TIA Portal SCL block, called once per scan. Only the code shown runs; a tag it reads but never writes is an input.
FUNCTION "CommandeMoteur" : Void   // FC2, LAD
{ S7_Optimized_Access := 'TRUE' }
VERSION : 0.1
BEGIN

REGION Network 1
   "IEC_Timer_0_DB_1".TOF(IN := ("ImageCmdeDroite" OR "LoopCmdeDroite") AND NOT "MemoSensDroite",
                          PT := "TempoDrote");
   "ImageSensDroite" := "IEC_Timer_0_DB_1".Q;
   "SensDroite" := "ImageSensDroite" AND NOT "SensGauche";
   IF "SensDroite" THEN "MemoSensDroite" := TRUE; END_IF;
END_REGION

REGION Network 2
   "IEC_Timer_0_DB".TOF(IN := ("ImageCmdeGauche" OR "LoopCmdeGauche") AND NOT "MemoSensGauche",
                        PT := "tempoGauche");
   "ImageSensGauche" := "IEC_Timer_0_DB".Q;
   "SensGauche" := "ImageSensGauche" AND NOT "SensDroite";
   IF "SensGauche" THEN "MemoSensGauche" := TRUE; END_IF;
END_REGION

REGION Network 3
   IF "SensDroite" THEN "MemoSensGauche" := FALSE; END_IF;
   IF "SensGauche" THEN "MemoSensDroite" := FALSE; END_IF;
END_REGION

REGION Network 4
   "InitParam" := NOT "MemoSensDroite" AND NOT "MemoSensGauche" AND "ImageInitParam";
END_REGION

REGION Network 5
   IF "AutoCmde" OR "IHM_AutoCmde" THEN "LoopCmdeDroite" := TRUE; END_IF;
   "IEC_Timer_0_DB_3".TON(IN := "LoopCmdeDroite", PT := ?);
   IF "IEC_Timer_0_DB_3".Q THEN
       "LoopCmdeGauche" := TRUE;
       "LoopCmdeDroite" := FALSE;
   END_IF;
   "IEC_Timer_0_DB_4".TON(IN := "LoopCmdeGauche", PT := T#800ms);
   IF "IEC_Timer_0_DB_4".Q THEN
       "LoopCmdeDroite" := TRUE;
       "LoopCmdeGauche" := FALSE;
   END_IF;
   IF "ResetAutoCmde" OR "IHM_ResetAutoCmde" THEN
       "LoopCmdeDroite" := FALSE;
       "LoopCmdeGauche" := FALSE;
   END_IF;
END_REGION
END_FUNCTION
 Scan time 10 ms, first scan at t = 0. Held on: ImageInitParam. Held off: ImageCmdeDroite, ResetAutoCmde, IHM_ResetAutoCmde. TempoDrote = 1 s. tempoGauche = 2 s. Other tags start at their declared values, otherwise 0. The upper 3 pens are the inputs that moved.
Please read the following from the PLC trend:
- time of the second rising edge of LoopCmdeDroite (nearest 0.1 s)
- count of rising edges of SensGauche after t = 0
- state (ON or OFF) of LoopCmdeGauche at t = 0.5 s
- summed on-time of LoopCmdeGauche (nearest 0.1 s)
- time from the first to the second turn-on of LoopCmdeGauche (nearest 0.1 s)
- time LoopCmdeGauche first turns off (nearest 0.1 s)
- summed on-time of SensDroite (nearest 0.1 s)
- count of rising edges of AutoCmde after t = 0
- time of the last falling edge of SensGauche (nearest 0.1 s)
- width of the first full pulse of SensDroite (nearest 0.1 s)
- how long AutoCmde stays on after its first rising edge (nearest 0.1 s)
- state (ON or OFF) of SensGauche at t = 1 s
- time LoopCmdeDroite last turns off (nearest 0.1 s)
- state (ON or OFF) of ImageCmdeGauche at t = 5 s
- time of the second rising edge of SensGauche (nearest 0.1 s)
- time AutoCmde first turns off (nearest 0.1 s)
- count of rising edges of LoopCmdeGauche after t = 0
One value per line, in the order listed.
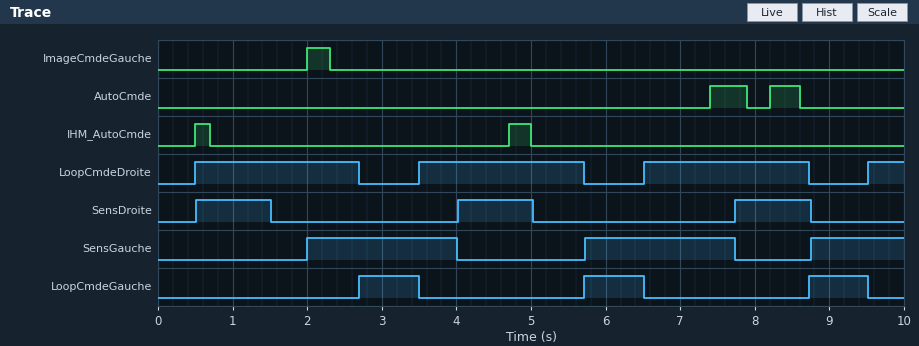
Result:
3.5 s
3
OFF
2.4 s
3.0 s
3.5 s
3.0 s
2
7.7 s
1.0 s
0.5 s
OFF
8.7 s
OFF
5.7 s
7.9 s
3
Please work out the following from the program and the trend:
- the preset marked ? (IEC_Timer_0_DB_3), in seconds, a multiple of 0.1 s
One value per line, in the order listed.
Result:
2.2 s
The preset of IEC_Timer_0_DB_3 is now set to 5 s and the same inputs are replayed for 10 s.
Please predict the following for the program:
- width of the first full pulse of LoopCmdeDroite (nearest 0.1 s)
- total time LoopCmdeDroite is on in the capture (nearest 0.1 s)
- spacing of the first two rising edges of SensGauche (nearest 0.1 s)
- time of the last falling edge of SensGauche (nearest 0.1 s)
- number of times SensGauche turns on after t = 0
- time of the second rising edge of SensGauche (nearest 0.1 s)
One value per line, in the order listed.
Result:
5.0 s
8.7 s
3.5 s
7.5 s
2
5.5 s
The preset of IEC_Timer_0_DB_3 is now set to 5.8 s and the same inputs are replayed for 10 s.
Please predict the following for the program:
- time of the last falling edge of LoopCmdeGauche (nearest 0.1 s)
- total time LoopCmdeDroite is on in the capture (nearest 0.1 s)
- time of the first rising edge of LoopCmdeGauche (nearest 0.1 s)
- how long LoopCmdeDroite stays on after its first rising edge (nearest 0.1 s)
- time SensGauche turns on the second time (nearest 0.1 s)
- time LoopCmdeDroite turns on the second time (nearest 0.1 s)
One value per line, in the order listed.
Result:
7.1 s
8.7 s
6.3 s
5.8 s
6.3 s
7.1 s
